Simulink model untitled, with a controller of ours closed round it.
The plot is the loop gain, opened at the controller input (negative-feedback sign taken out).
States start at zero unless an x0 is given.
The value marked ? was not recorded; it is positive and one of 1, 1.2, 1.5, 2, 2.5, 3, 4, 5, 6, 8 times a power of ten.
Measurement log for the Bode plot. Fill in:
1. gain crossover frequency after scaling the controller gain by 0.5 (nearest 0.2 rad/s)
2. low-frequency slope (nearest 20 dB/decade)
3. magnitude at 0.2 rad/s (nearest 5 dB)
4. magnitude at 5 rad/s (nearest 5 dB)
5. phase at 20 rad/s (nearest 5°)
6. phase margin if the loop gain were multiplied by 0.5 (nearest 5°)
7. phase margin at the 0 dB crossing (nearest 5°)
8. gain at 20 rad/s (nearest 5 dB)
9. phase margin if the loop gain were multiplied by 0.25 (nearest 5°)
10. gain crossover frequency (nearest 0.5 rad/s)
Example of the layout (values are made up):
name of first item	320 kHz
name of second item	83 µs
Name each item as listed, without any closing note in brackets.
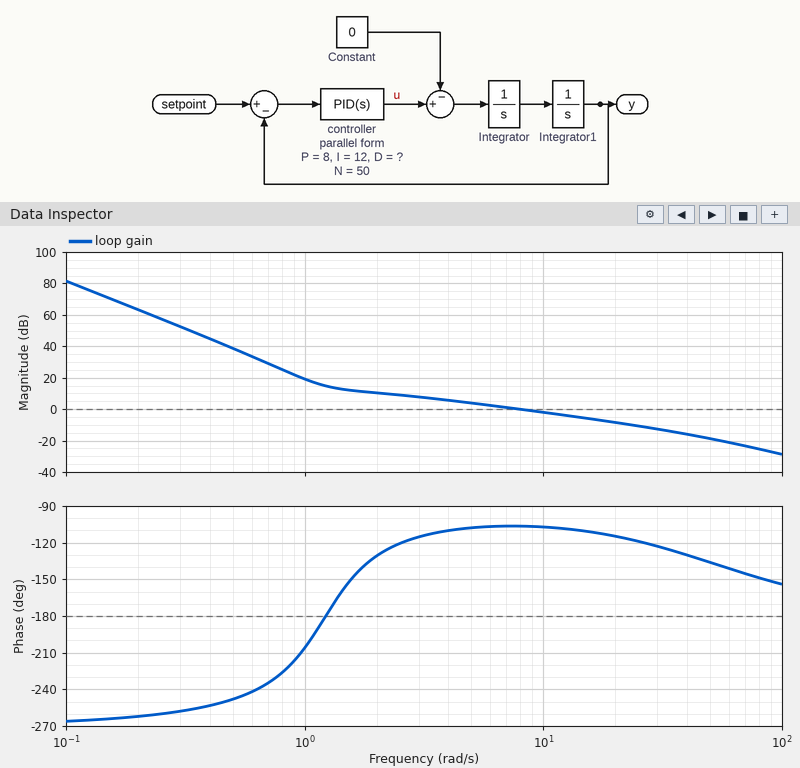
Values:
gain crossover frequency after scaling the controller gain by 0.5	3.8 rad/s
low-frequency slope	-60 dB/decade
magnitude at 0.2 rad/s	65 dB
magnitude at 5 rad/s	5 dB
phase at 20 rad/s	-115°
phase margin if the loop gain were multiplied by 0.5	70°
phase margin at the 0 dB crossing	75°
gain at 20 rad/s	-10 dB
phase margin if the loop gain were multiplied by 0.25	30°
gain crossover frequency	8.0 rad/s
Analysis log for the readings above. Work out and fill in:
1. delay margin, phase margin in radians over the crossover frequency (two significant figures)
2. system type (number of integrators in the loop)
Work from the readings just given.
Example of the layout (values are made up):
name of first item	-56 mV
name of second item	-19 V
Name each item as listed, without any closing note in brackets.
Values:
delay margin, phase margin in radians over the crossover frequency	0.16 s
system type	3
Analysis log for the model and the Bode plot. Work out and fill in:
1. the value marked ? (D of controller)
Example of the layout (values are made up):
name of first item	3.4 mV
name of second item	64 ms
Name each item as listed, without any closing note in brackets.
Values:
the value marked ?	8
